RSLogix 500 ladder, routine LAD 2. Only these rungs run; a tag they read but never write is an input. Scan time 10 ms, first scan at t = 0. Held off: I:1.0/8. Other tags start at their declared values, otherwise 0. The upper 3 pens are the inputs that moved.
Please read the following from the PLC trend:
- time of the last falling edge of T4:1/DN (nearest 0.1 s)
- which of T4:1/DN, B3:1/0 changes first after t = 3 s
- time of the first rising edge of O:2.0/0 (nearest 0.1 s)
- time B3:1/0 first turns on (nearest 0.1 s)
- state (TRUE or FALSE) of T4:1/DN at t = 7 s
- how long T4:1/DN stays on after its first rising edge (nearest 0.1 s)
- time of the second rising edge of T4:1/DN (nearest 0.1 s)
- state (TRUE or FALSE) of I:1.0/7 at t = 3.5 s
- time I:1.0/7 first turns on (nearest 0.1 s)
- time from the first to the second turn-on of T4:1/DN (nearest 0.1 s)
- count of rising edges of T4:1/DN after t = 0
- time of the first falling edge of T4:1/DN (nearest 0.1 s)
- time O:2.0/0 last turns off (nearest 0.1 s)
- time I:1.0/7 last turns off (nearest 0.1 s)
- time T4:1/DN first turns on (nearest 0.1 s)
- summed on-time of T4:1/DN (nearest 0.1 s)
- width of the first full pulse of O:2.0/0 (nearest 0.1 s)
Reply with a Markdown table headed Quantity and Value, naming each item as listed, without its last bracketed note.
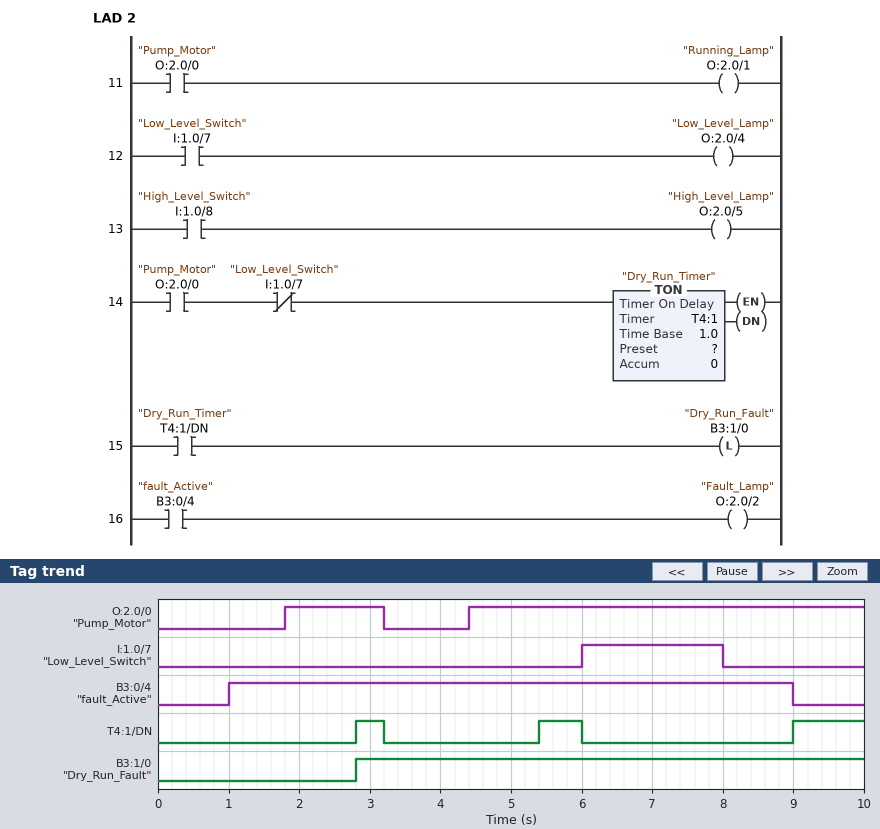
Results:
| Quantity | Value |
|---|---|
| time of the last falling edge of T4:1/DN | 6.0 s |
| which of T4:1/DN, B3:1/0 changes first after t = 3 s | T4:1/DN |
| time of the first rising edge of O:2.0/0 | 1.8 s |
| time B3:1/0 first turns on | 2.8 s |
| state (TRUE or FALSE) of T4:1/DN at t = 7 s | FALSE |
| how long T4:1/DN stays on after its first rising edge | 0.4 s |
| time of the second rising edge of T4:1/DN | 5.4 s |
| state (TRUE or FALSE) of I:1.0/7 at t = 3.5 s | FALSE |
| time I:1.0/7 first turns on | 6.0 s |
| time from the first to the second turn-on of T4:1/DN | 2.6 s |
| count of rising edges of T4:1/DN after t = 0 | 3 |
| time of the first falling edge of T4:1/DN | 3.2 s |
| time O:2.0/0 last turns off | 3.2 s |
| time I:1.0/7 last turns off | 8.0 s |
| time T4:1/DN first turns on | 2.8 s |
| summed on-time of T4:1/DN | 2.0 s |
| width of the first full pulse of O:2.0/0 | 1.4 s |
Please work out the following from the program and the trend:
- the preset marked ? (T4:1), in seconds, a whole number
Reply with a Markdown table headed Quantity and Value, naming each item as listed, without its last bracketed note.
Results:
| Quantity | Value |
|---|---|
| the preset marked ? (T4:1), in seconds, a whole number | 1 s |
